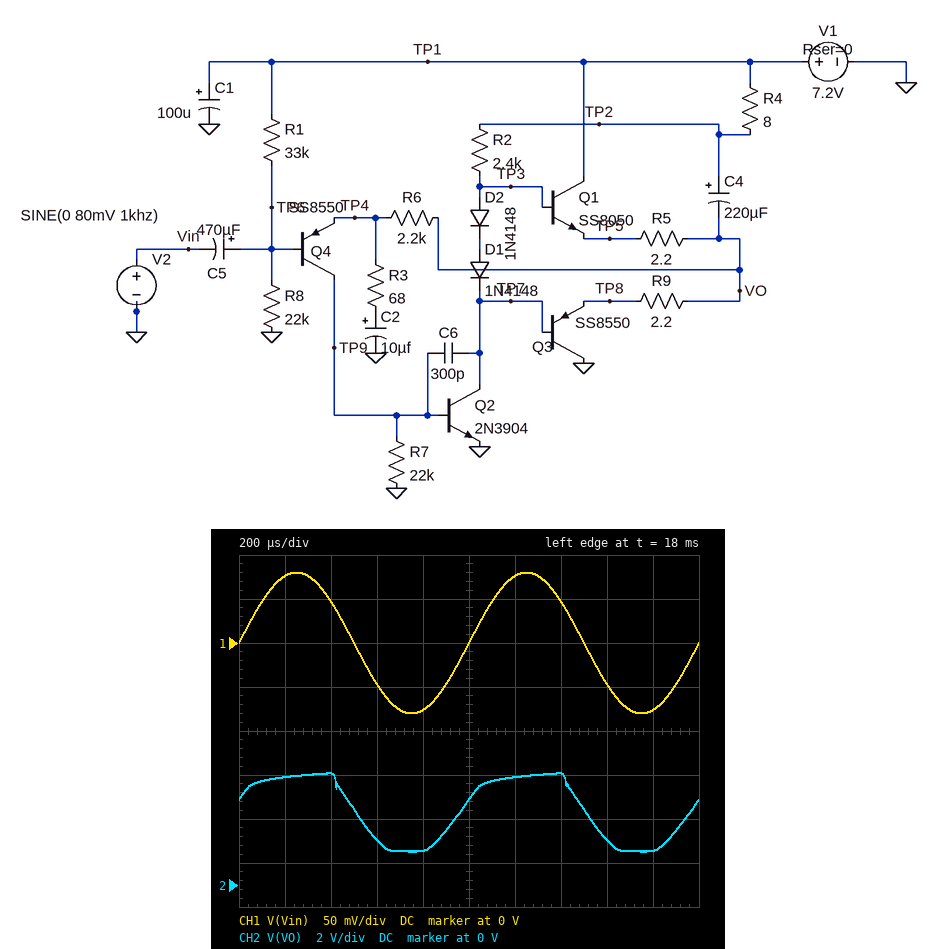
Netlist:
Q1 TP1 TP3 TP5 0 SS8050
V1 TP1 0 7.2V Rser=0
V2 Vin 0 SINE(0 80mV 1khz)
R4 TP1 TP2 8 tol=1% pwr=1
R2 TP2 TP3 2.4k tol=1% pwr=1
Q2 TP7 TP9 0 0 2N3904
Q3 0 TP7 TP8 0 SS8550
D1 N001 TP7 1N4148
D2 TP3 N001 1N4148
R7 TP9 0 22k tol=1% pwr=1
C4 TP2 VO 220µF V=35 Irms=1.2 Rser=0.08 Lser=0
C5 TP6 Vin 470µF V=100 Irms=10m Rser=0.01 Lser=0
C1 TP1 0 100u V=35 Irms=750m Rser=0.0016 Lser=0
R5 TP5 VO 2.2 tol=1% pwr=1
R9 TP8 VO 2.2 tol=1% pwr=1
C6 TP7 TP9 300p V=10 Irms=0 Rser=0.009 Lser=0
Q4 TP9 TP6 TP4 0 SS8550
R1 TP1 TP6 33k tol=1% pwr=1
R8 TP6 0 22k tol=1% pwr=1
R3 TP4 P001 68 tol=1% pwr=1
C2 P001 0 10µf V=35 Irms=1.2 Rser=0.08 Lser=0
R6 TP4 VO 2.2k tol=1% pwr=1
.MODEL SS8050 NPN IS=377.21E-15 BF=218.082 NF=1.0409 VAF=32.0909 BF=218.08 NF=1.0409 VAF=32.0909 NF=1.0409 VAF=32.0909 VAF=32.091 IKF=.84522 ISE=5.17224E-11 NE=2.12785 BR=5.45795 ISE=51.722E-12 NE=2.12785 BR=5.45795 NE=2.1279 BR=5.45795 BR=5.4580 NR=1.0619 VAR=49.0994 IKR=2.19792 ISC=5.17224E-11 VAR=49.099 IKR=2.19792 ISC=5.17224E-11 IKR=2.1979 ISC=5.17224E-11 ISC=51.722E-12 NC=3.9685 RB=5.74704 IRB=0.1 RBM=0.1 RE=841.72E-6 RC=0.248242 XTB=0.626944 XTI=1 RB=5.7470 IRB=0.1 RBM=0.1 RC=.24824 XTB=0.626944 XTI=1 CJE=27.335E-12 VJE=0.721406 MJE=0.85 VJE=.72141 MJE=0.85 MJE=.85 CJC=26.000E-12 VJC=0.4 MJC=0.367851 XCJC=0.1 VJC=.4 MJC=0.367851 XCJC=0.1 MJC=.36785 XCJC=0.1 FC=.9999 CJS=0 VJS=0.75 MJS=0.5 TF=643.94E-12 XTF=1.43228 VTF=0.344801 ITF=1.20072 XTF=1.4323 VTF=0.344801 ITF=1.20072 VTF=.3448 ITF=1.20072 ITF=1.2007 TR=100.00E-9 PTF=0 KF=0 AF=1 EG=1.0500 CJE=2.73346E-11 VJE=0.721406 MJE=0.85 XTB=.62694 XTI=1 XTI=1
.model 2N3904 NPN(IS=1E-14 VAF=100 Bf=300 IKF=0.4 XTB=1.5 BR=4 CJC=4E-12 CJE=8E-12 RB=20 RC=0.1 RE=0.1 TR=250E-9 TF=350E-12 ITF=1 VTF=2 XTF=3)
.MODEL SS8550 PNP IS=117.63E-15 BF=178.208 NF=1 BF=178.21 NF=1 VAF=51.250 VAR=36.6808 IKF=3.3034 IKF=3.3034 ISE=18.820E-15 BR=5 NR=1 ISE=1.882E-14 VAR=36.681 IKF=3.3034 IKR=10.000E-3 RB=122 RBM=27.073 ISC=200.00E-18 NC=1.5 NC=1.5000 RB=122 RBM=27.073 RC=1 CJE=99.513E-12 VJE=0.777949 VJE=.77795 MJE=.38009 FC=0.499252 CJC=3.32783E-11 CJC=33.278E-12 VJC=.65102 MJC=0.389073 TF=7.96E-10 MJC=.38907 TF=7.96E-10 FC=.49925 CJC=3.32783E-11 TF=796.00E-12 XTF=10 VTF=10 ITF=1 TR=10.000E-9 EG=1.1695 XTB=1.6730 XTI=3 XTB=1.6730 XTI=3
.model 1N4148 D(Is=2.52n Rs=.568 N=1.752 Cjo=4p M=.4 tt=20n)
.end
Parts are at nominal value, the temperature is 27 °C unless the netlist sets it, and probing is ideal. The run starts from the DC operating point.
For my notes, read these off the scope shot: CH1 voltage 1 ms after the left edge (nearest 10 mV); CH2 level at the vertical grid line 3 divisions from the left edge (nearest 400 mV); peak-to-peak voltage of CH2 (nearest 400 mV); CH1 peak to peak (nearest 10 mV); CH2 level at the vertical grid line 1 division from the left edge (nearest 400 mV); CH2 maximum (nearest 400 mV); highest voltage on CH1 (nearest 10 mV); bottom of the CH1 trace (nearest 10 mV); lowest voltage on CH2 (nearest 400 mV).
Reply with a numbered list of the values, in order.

1. 0 V
2. 2.0 V
3. 3.6 V
4. 160 mV
5. 4.8 V
6. 5.2 V
7. 80 mV
8. -80 mV
9. 1.6 V
